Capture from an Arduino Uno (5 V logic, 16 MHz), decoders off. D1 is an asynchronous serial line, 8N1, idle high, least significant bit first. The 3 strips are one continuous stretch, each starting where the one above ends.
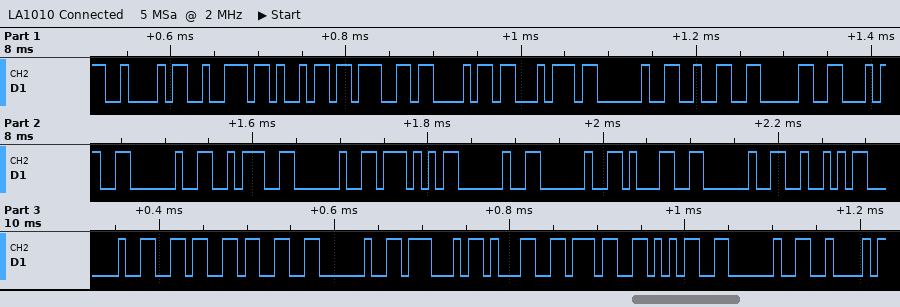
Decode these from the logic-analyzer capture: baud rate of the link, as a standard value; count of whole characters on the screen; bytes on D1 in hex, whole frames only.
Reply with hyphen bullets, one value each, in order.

- 115200 baud
- 29
- 42 72 69 67 68 74 20 32 30 34 20 3A 20 57 20 20 31 20 52 20 36 33 20 47 31 37 35 20 42
